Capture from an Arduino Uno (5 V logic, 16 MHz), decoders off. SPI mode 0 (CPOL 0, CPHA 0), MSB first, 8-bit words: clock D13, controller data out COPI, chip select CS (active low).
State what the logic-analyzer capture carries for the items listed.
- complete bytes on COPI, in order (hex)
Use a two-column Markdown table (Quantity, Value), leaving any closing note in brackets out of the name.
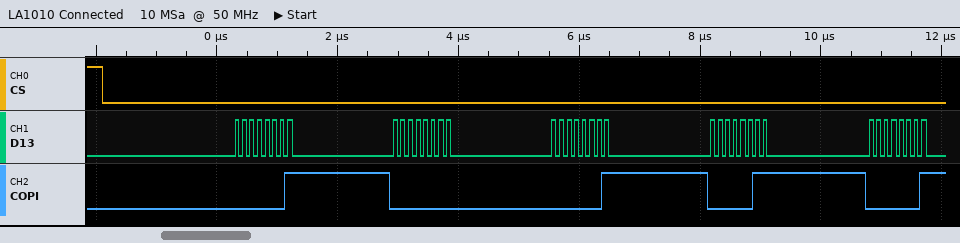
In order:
| Quantity | Value |
|---|---|
| complete bytes on COPI, in order | 01 00 01 03 01 |
